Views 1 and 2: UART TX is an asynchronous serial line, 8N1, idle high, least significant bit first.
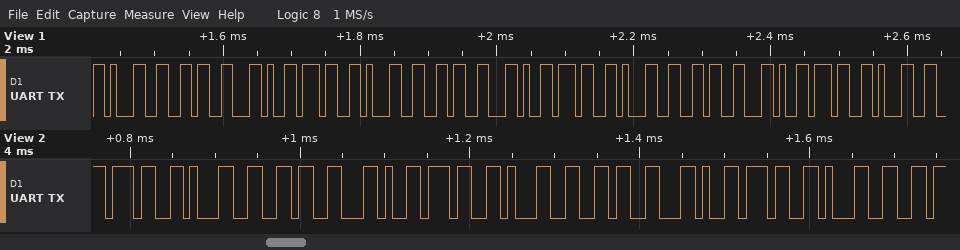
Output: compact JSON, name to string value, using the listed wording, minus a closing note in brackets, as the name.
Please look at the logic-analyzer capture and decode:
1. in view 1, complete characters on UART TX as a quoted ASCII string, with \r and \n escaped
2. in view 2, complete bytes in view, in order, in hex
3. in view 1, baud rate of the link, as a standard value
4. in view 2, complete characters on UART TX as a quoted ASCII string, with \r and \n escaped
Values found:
{"in view 1, complete characters on UART TX as a quoted ASCII string, with \\r and \\n escaped": "\"16,716,716,71\"", "in view 2, complete bytes in view, in order, in hex": "0x37 0x31 0x36 0x2C 0x37 0x31 0x36 0x2C 0x37 0x31", "in view 1, baud rate of the link, as a standard value": "115200 baud", "in view 2, complete characters on UART TX as a quoted ASCII string, with \\r and \\n escaped": "\"716,716,71\""}
